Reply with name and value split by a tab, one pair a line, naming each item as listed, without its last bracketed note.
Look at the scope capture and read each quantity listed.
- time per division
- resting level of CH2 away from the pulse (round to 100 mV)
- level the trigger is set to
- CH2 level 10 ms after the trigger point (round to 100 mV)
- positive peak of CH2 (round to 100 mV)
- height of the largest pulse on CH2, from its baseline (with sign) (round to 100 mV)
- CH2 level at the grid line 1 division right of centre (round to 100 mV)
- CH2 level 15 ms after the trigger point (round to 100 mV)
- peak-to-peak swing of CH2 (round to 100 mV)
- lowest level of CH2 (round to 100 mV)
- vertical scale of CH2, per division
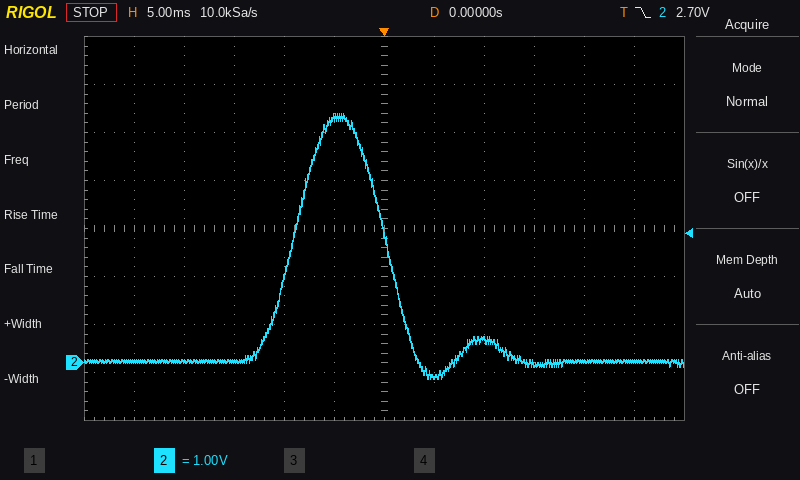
time per division	5 ms
resting level of CH2 away from the pulse	0.0 V
level the trigger is set to	2.70 V
CH2 level 10 ms after the trigger point	500 mV
positive peak of CH2	5.2 V
height of the largest pulse on CH2, from its baseline (with sign)	+5.2 V
CH2 level at the grid line 1 division right of centre	-300 mV
CH2 level 15 ms after the trigger point	0.0 V
peak-to-peak swing of CH2	5.5 V
lowest level of CH2	-300 mV
vertical scale of CH2, per division	1 V
